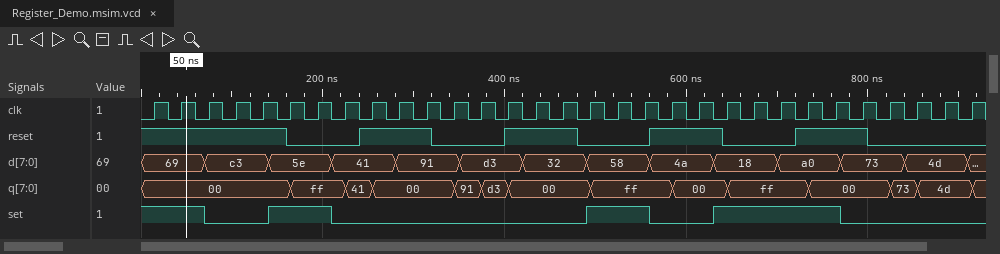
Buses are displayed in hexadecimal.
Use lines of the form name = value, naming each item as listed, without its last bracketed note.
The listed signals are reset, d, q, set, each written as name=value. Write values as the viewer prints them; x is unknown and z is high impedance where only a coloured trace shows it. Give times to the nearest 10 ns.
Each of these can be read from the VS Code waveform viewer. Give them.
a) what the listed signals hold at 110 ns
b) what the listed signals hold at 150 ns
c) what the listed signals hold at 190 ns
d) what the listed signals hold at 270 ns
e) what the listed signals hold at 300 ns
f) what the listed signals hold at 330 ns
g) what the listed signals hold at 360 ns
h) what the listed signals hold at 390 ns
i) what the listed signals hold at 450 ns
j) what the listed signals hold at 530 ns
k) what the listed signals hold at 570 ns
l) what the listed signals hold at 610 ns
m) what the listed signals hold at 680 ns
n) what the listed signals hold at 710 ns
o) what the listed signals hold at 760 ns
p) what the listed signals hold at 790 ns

what the listed signals hold at 110 ns = reset=1, d=c3, q=00, set=0
what the listed signals hold at 150 ns = reset=1, d=5e, q=00, set=1
what the listed signals hold at 190 ns = reset=0, d=5e, q=ff, set=1
what the listed signals hold at 270 ns = reset=1, d=41, q=00, set=0
what the listed signals hold at 300 ns = reset=1, d=91, q=00, set=0
what the listed signals hold at 330 ns = reset=0, d=91, q=00, set=0
what the listed signals hold at 360 ns = reset=0, d=d3, q=91, set=0
what the listed signals hold at 390 ns = reset=0, d=d3, q=d3, set=0
what the listed signals hold at 450 ns = reset=1, d=32, q=00, set=0
what the listed signals hold at 530 ns = reset=0, d=58, q=ff, set=1
what the listed signals hold at 570 ns = reset=1, d=4a, q=ff, set=0
what the listed signals hold at 610 ns = reset=1, d=4a, q=00, set=0
what the listed signals hold at 680 ns = reset=0, d=18, q=ff, set=1
what the listed signals hold at 710 ns = reset=0, d=a0, q=ff, set=1
what the listed signals hold at 760 ns = reset=1, d=a0, q=00, set=1
what the listed signals hold at 790 ns = reset=1, d=73, q=00, set=0
